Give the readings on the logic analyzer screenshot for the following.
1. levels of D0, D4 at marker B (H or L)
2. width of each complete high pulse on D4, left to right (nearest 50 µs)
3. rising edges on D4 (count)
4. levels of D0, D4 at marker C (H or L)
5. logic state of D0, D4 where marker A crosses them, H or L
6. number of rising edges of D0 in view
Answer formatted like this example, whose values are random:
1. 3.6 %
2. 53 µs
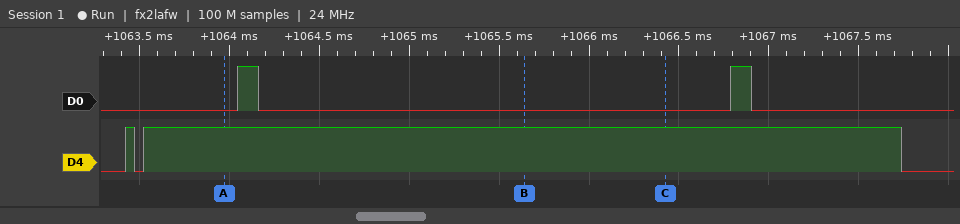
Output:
1. D0=L, D4=H
2. 50 µs, 4200 µs
3. 2
4. D0=L, D4=H
5. D0=L, D4=H
6. 2
